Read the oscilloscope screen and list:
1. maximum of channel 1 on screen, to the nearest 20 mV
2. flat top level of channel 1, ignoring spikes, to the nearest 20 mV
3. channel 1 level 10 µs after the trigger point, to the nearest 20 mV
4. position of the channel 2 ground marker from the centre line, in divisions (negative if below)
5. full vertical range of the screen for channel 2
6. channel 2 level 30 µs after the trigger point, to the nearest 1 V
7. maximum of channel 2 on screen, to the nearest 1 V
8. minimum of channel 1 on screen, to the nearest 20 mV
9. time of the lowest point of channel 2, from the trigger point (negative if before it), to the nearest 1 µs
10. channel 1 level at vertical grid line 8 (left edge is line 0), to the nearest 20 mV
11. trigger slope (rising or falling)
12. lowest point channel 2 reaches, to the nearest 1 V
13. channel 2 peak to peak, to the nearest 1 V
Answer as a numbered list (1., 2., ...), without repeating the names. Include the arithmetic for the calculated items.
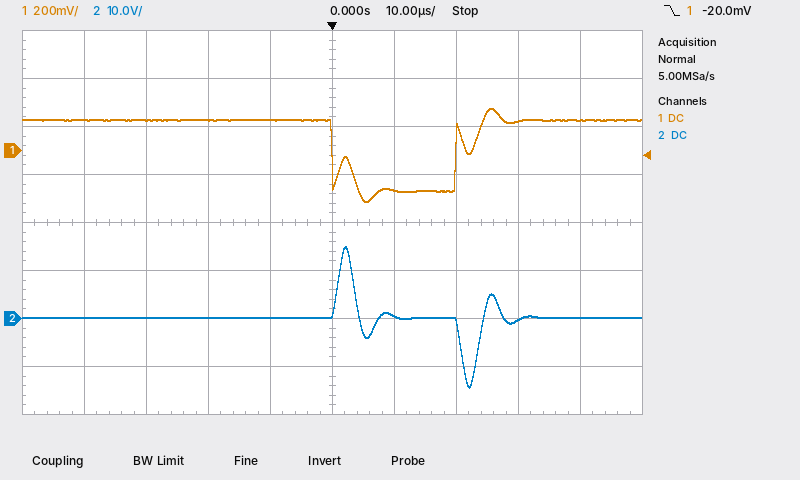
1. 180 mV
2. 120 mV
3. -160 mV
4. -2.0 div
5. 80 V
6. 0 V
7. 15 V
8. -220 mV
9. +22 µs
10. 120 mV
11. falling
12. -14 V
13. 15 V − (-14 V) = 29 V
